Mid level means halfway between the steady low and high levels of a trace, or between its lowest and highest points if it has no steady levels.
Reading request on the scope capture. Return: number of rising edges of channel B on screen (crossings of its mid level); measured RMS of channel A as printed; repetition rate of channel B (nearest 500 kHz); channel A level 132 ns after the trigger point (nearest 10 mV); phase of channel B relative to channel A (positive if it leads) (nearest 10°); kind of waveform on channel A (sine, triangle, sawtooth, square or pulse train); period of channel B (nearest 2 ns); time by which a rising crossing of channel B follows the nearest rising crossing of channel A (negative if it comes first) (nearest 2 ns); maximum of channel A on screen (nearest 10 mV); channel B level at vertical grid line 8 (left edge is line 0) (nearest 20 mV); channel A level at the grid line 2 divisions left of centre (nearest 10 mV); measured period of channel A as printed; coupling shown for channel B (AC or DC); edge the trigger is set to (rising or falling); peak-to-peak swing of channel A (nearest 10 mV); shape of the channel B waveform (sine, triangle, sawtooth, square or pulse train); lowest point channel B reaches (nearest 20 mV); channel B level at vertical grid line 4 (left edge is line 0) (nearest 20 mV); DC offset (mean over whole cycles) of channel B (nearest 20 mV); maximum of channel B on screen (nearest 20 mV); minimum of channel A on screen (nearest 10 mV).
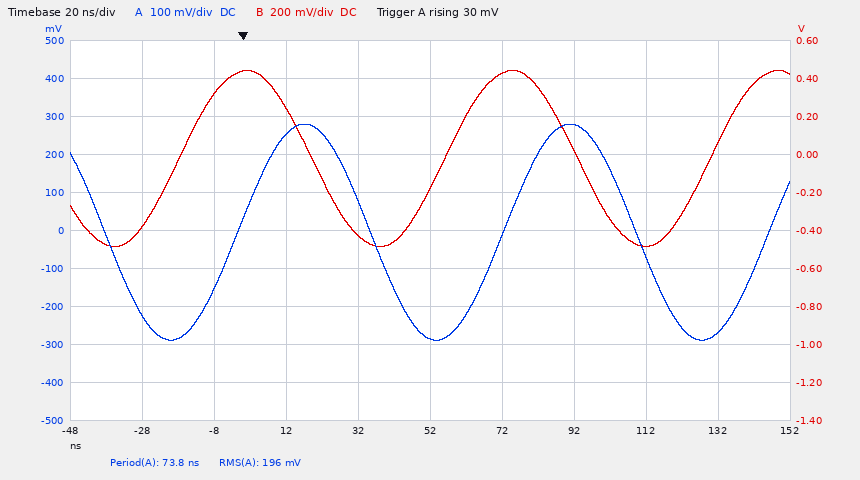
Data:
3
196 mV
13.5 MHz
-270 mV
+80°
sine
74 ns
-16 ns
280 mV
-480 mV
250 mV
73.8 ns
DC
rising
570 mV
sine
-480 mV
-420 mV
-20 mV
440 mV
-290 mV
